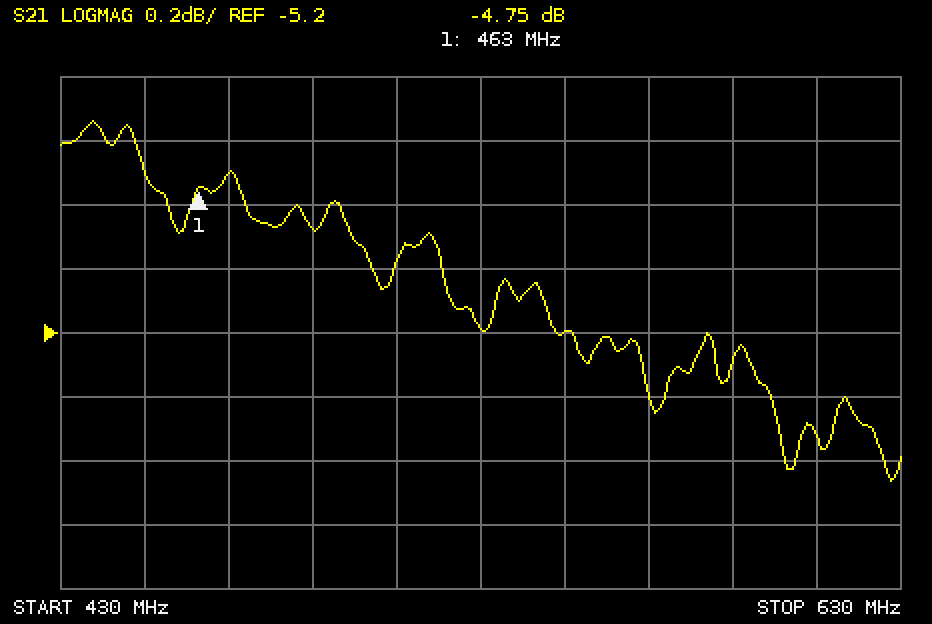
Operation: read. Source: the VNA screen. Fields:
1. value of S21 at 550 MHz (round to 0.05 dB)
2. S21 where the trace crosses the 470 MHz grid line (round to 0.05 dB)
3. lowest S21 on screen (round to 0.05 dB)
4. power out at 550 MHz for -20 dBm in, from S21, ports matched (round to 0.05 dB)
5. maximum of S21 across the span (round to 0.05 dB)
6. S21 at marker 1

-5.20 dB
-4.70 dB
-5.65 dB
-25.20 dBm
-4.55 dB
-4.75 dB
